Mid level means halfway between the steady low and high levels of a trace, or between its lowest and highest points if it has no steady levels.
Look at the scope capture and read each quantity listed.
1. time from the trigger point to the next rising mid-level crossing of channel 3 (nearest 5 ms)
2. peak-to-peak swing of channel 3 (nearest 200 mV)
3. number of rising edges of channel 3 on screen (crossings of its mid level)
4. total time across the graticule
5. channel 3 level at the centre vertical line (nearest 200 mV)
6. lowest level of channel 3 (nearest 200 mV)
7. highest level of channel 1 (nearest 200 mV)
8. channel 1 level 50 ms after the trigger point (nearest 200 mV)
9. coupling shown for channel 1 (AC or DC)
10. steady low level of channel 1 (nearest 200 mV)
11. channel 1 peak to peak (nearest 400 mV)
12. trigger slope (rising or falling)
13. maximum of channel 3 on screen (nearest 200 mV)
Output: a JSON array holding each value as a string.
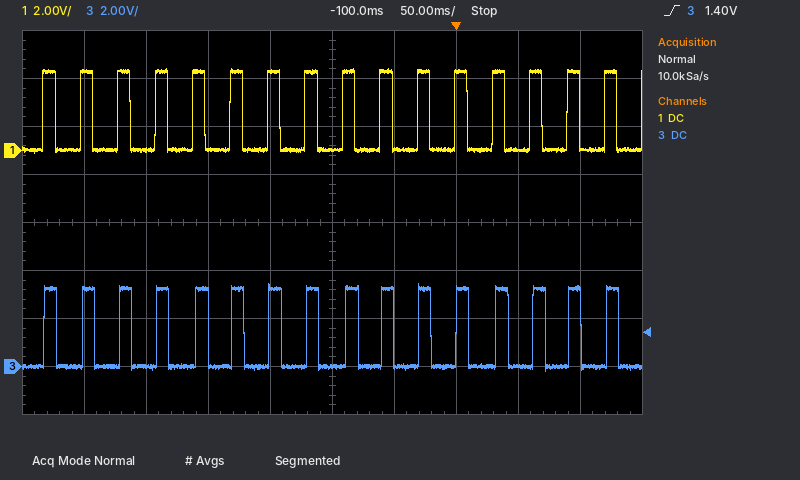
["30 ms", "3.6 V", "16", "500 ms", "0.0 V", "-200 mV", "3.4 V", "0.0 V", "DC", "0.0 V", "3.6 V", "rising", "3.4 V"]
